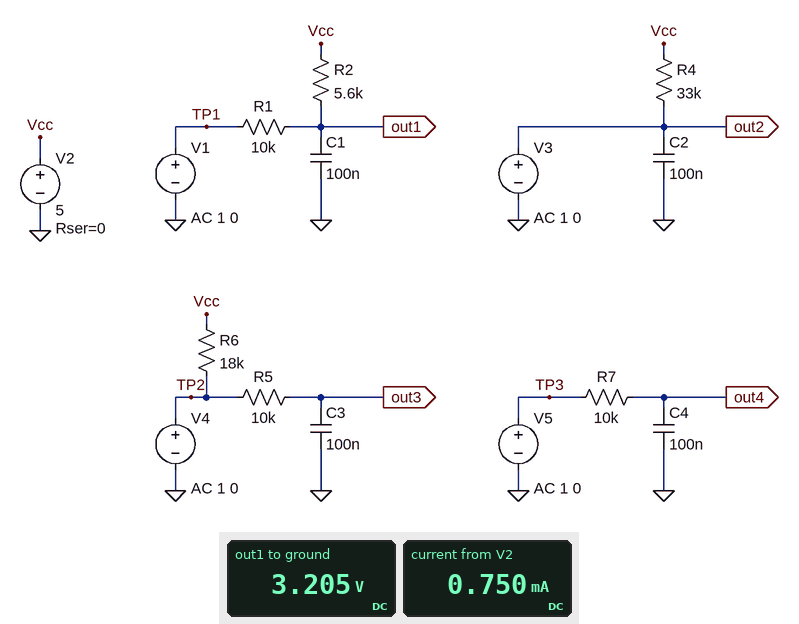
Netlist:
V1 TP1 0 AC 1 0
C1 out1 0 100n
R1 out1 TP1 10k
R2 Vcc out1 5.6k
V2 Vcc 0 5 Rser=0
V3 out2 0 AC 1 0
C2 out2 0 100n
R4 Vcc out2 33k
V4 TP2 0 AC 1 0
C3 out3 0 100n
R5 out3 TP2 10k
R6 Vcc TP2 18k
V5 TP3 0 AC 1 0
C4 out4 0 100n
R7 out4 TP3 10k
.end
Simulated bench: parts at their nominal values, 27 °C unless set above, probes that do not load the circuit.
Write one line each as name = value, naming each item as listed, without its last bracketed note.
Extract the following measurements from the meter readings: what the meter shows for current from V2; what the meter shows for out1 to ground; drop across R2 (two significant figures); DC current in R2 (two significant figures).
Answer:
what the meter shows for current from V2 = 0.750 mA
what the meter shows for out1 to ground = 3.205 V
drop across R2 = 1.8 V
DC current in R2 = 320 µA
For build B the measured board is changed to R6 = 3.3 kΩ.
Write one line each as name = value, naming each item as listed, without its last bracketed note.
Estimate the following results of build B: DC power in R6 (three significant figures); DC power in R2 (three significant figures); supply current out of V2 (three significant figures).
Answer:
DC power in R6 = 7.58 mW
DC power in R2 = 575 µW
supply current out of V2 = 1.99 mA
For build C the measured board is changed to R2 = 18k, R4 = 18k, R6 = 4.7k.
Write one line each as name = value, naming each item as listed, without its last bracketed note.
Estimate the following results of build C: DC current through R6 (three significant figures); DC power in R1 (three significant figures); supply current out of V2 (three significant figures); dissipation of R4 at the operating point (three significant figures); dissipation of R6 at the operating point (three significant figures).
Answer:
DC current through R6 = 1.06 mA
DC power in R1 = 319 µW
supply current out of V2 = 1.52 mA
dissipation of R4 at the operating point = 1.39 mW
dissipation of R6 at the operating point = 5.32 mW
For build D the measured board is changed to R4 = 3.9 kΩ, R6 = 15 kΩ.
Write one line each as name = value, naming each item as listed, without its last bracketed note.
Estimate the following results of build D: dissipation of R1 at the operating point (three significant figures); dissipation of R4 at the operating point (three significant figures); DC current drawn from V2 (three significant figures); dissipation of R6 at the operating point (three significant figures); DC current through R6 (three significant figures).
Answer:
dissipation of R1 at the operating point = 1.03 mW
dissipation of R4 at the operating point = 6.41 mW
DC current drawn from V2 = 1.94 mA
dissipation of R6 at the operating point = 1.67 mW
DC current through R6 = 333 µA
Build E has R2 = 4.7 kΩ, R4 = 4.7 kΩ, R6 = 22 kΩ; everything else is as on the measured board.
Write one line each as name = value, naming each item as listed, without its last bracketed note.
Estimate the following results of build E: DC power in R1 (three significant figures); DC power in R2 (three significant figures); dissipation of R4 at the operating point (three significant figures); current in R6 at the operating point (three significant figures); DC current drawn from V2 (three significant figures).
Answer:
DC power in R1 = 1.16 mW
DC power in R2 = 544 µW
dissipation of R4 at the operating point = 5.32 mW
current in R6 at the operating point = 227 µA
DC current drawn from V2 = 1.63 mA
